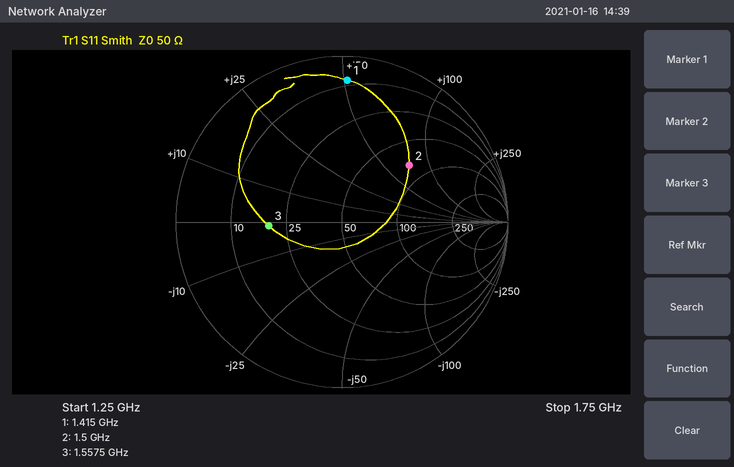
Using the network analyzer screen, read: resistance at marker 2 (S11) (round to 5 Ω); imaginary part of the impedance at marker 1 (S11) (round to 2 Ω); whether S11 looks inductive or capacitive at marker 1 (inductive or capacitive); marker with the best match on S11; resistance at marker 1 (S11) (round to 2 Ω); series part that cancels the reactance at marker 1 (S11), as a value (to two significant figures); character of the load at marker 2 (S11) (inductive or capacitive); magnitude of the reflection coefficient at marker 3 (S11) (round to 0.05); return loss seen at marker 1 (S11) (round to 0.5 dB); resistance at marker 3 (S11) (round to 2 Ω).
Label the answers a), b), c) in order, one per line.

a) 75 Ω
b) +52 Ω
c) inductive
d) marker 3
e) 8 Ω
f) 2.2 pF
g) inductive
h) 0.45
i) 1.5 dB
j) 20 Ω
